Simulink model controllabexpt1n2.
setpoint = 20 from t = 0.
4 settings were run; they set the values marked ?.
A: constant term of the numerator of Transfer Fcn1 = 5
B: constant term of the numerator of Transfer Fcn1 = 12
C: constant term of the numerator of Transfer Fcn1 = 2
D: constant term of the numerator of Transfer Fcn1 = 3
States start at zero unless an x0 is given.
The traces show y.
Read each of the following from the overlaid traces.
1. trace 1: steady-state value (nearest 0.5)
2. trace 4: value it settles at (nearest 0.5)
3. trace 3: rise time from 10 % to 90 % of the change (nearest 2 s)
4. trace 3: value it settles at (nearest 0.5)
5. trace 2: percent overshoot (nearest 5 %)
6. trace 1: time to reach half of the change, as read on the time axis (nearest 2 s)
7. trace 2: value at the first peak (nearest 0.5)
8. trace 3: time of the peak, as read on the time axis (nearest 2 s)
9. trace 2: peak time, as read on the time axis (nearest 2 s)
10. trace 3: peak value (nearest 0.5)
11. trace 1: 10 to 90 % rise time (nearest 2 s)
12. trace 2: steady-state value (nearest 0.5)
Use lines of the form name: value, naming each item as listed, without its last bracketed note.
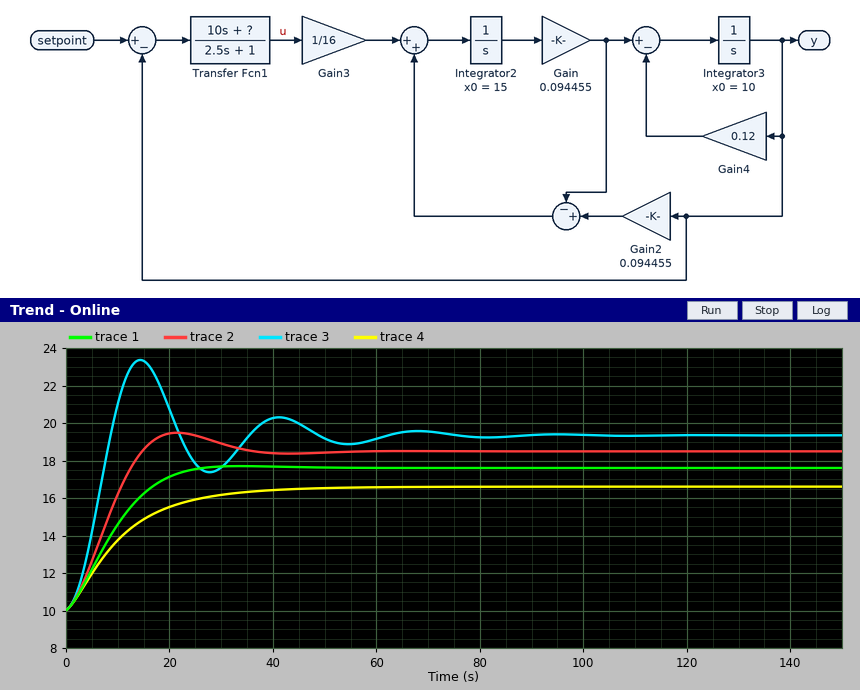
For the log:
trace 1: steady-state value: 17.5
trace 4: value it settles at: 16.5
trace 3: rise time from 10 % to 90 % of the change: 6 s
trace 3: value it settles at: 19.5
trace 2: percent overshoot: 10 %
trace 1: time to reach half of the change, as read on the time axis: 8 s
trace 2: value at the first peak: 19.5
trace 3: time of the peak, as read on the time axis: 14 s
trace 2: peak time, as read on the time axis: 22 s
trace 3: peak value: 23.5
trace 1: 10 to 90 % rise time: 16 s
trace 2: steady-state value: 18.5
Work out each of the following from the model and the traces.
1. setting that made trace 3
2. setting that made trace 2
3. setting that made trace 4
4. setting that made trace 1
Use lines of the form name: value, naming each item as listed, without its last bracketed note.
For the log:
setting that made trace 3: B
setting that made trace 2: A
setting that made trace 4: C
setting that made trace 1: D
